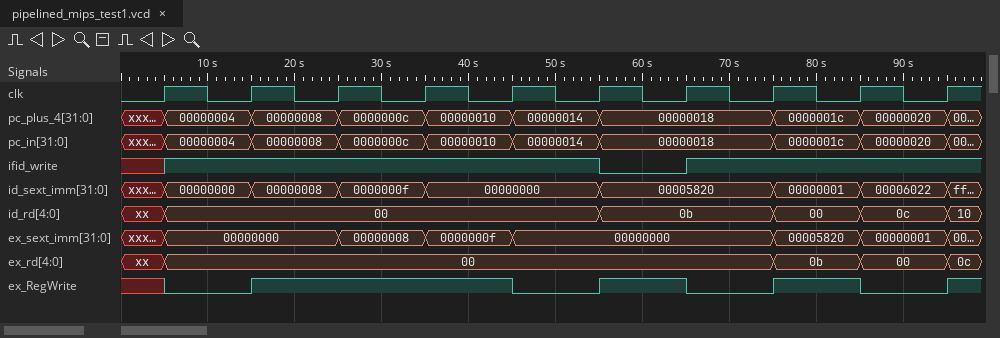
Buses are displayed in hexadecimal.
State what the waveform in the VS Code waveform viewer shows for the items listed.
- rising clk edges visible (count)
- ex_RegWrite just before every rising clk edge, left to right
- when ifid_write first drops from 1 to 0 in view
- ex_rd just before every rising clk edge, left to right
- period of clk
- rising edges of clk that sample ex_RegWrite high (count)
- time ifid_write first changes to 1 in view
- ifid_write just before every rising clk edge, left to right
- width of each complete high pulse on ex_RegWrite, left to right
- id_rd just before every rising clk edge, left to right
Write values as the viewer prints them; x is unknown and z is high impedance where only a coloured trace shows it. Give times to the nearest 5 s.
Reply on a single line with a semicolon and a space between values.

10; x 0 1 1 1 0 1 0 1 0; 55 s; xx, 00, 00, 00, 00, 00, 00, 00, 0b, 00; 10 s; 5; 5 s; x 1 1 1 1 1 0 1 1 1; 30 s, 10 s, 10 s; xx, 00, 00, 00, 00, 00, 0b, 0b, 00, 0c
